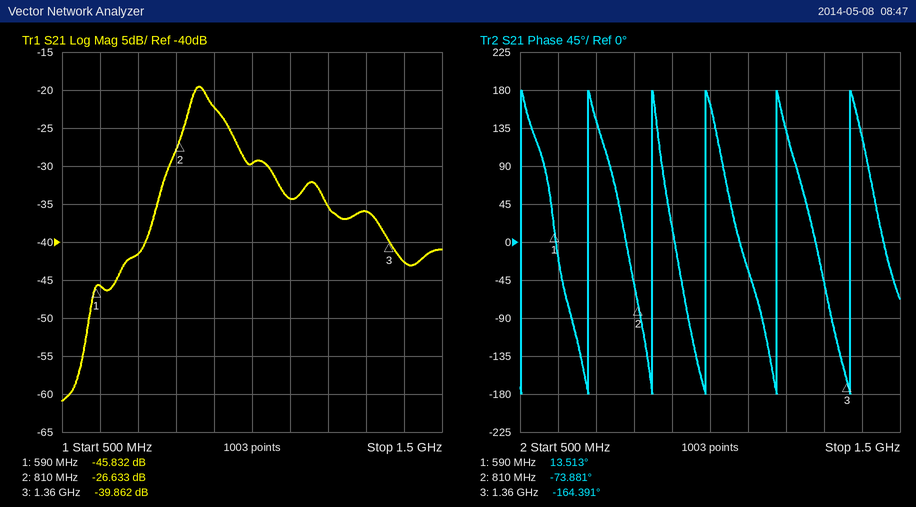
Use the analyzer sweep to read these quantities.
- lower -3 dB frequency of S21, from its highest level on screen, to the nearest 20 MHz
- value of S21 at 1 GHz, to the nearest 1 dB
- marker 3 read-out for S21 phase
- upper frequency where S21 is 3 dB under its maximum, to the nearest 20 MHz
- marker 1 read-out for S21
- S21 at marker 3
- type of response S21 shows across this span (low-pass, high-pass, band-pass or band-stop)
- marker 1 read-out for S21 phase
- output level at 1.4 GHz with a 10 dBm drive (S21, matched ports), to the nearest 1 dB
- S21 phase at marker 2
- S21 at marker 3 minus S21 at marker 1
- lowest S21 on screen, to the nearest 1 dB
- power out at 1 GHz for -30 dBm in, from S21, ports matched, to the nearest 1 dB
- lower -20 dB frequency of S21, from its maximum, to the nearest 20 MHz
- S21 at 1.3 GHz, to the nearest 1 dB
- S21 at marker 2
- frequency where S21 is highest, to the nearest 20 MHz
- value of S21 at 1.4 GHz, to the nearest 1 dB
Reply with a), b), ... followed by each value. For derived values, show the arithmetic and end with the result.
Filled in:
a) 840 MHz
b) -30 dB
c) -164.391°
d) 900 MHz
e) -45.832 dB
f) -39.862 dB
g) band-pass
h) 13.513°
i) 10 dBm + (-43 dB) = -33 dBm
j) -73.881°
k) -39.862 − (-45.832) = 5.970 dB
l) -61 dB
m) -30 dBm + (-30 dB) = -60 dBm
n) 720 MHz
o) -36 dB
p) -26.633 dB
q) 860 MHz
r) -43 dB
